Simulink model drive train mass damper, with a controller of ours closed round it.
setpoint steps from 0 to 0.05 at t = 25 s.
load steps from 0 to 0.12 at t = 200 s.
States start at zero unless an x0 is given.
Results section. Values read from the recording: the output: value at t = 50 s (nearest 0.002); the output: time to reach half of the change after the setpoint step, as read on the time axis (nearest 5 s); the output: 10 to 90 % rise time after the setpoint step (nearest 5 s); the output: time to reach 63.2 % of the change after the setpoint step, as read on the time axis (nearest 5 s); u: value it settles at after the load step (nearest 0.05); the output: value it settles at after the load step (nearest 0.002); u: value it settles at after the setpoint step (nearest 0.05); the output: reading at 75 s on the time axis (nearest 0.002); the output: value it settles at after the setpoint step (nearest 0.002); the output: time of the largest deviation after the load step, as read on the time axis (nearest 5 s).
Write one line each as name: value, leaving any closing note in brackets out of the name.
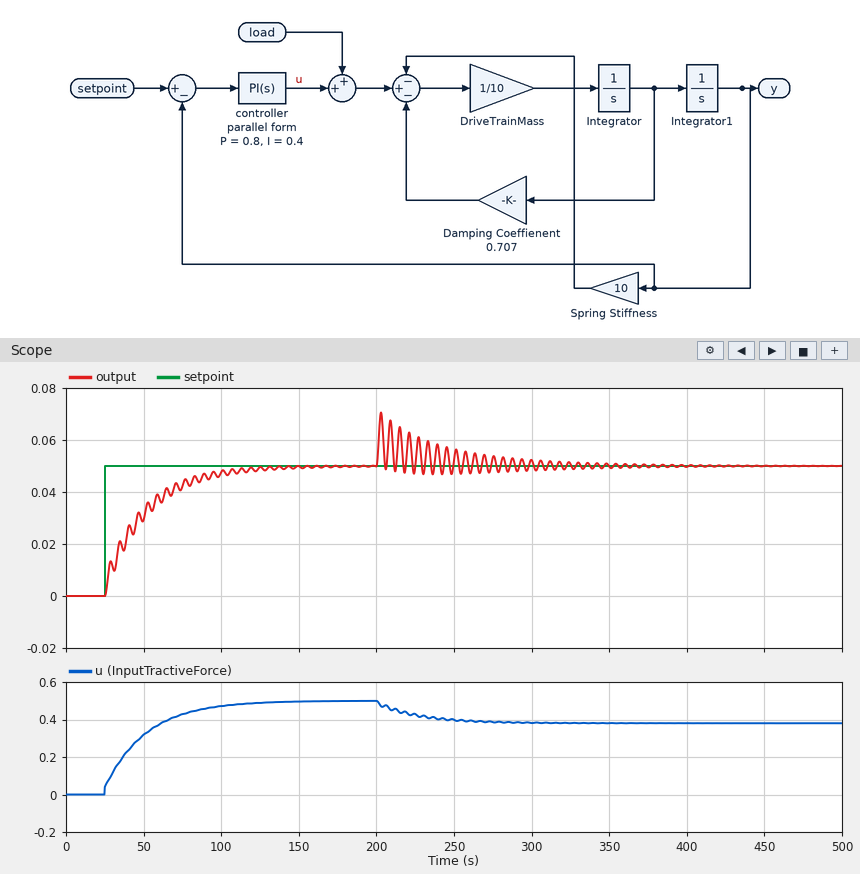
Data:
the output: value at t = 50 s: 0.030
the output: time to reach half of the change after the setpoint step, as read on the time axis: 40 s
the output: 10 to 90 % rise time after the setpoint step: 55 s
the output: time to reach 63.2 % of the change after the setpoint step, as read on the time axis: 45 s
u: value it settles at after the load step: 0.40
the output: value it settles at after the load step: 0.050
u: value it settles at after the setpoint step: 0.50
the output: reading at 75 s on the time axis: 0.042
the output: value it settles at after the setpoint step: 0.050
the output: time of the largest deviation after the load step, as read on the time axis: 205 s
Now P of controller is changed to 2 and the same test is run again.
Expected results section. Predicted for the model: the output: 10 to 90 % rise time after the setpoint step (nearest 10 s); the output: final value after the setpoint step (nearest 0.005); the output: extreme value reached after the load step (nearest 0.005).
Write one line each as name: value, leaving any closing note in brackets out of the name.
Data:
the output: 10 to 90 % rise time after the setpoint step: 50 s
the output: final value after the setpoint step: 0.050
the output: extreme value reached after the load step: 0.070
